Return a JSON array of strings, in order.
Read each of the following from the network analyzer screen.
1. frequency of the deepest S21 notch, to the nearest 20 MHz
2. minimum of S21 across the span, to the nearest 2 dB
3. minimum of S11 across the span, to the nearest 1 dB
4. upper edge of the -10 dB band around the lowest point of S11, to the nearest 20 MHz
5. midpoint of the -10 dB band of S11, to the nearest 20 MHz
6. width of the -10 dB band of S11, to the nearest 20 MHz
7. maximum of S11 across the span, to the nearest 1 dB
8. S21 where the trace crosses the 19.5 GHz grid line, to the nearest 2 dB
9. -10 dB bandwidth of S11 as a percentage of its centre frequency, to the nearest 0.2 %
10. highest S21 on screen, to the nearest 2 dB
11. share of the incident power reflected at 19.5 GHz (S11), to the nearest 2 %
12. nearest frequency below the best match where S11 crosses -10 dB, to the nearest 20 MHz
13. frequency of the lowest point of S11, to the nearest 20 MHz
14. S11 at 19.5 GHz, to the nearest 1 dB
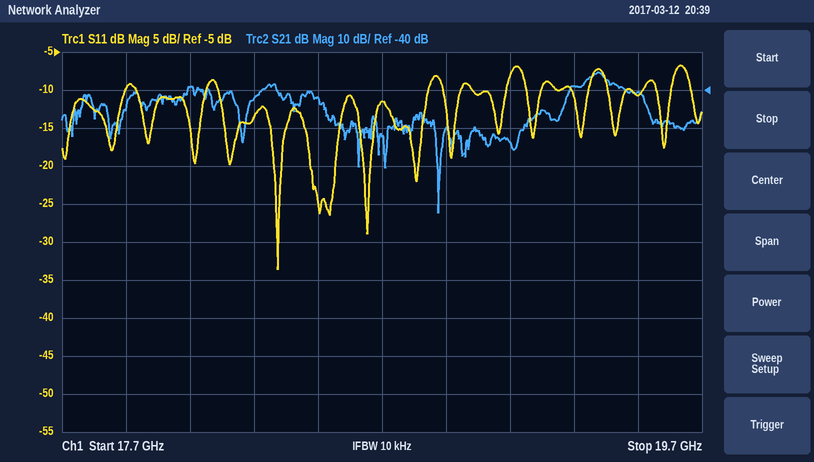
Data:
["18.88 GHz", "-72 dB", "-34 dB", "18.84 GHz", "18.52 GHz", "660 MHz", "-7 dB", "-40 dB", "3.6 %", "-36 dB", "8 %", "18.18 GHz", "18.38 GHz", "-11 dB"]
